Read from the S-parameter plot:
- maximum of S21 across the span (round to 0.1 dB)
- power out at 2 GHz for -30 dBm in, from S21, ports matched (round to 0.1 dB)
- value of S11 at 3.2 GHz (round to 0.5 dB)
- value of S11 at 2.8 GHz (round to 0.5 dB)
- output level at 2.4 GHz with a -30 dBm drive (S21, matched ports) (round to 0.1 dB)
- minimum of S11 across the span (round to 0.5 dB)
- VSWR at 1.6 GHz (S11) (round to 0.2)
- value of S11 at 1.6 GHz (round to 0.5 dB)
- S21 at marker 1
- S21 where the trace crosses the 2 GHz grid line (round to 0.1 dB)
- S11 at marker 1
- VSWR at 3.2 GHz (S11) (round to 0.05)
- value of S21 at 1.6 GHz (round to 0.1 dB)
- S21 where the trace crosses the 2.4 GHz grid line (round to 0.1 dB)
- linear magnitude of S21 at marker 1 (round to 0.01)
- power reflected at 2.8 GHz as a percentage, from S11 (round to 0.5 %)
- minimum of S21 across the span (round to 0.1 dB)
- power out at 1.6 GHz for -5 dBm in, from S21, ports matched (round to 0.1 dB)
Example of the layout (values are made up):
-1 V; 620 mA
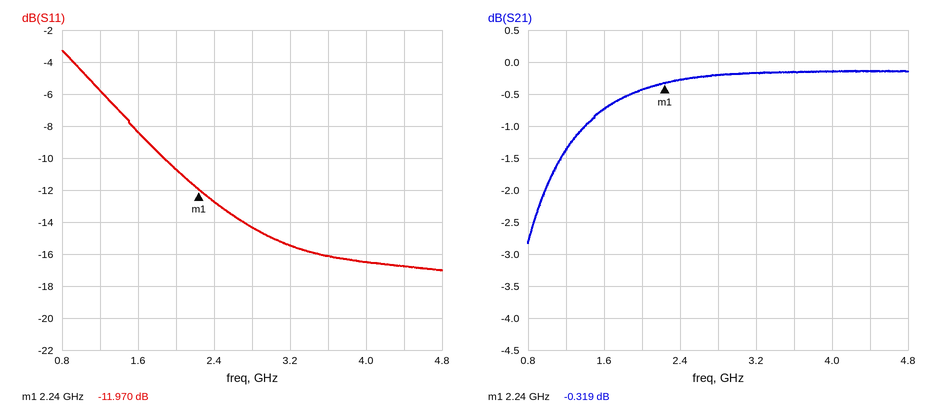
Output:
-0.1 dB; -30.4 dBm; -15.5 dB; -14.5 dB; -30.3 dBm; -17.0 dB; 2.2; -8.5 dB; -0.319 dB; -0.4 dB; -11.970 dB; 1.40; -0.7 dB; -0.3 dB; 0.96; 3.5 %; -2.8 dB; -5.7 dBm
